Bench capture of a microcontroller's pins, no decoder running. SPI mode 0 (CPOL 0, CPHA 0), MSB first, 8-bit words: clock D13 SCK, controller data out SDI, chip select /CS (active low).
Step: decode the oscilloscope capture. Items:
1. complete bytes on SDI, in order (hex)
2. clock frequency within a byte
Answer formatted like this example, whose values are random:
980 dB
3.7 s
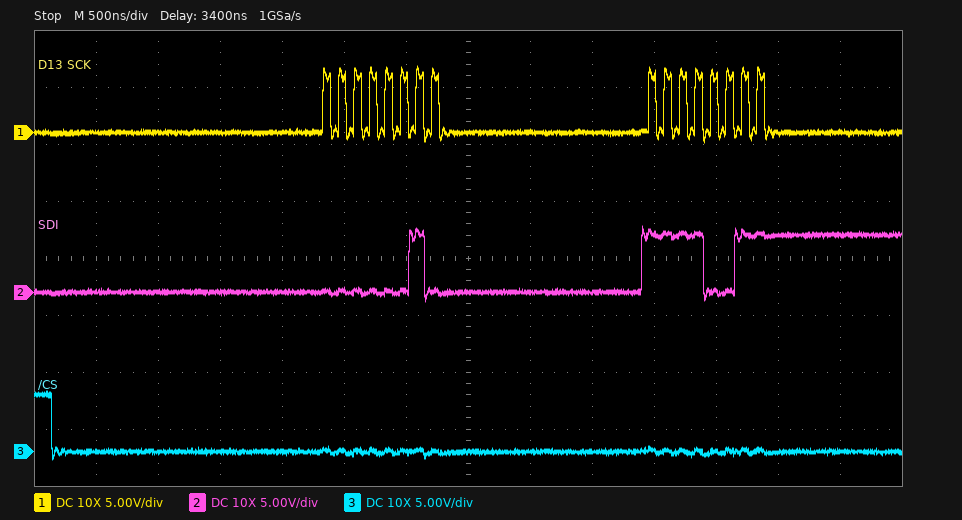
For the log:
02 F3
8 MHz
